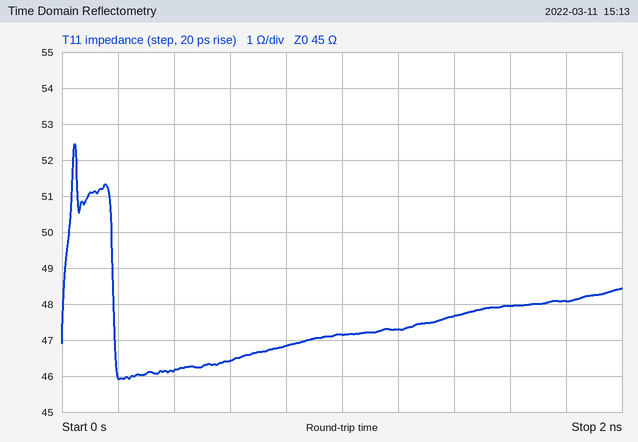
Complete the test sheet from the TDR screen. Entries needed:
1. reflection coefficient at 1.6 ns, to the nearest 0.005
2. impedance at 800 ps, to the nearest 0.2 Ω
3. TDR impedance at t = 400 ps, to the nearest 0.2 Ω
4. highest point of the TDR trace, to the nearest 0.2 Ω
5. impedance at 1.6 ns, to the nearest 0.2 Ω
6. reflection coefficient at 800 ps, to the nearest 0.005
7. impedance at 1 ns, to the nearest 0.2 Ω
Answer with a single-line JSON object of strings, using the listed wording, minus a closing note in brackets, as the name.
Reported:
{"reflection coefficient at 1.6 ns, to the nearest 0.005": "+0.030", "impedance at 800 ps, to the nearest 0.2 Ω": "46.8 Ω", "TDR impedance at t = 400 ps, to the nearest 0.2 Ω": "46.2 Ω", "highest point of the TDR trace, to the nearest 0.2 Ω": "52.4 Ω", "impedance at 1.6 ns, to the nearest 0.2 Ω": "48.0 Ω", "reflection coefficient at 800 ps, to the nearest 0.005": "+0.020", "impedance at 1 ns, to the nearest 0.2 Ω": "47.2 Ω"}
